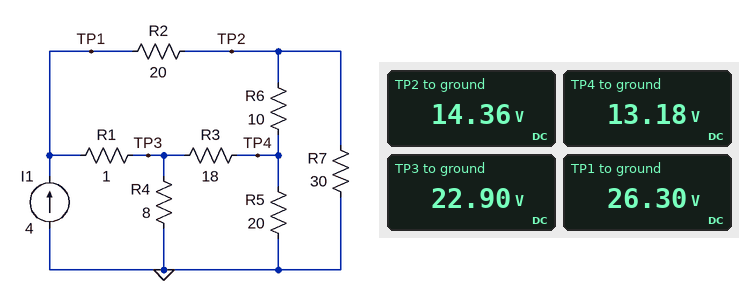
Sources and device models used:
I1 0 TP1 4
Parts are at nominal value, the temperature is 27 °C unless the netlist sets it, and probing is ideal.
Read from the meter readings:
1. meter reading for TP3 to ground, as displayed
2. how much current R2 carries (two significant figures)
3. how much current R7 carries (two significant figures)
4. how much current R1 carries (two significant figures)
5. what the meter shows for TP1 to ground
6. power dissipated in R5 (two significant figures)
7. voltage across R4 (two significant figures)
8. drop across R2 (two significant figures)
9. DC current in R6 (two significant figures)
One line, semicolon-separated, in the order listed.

22.90 V; 600 mA; 480 mA; 3.4 A; 26.30 V; 8.7 W; 23 V; 12 V; 120 mA
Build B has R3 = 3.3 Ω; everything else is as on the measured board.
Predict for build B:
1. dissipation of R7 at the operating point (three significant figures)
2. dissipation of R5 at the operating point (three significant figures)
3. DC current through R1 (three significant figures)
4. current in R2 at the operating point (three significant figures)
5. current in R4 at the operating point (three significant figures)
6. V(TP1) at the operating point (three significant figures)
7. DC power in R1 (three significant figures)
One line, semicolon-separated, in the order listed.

8.68 W; 15.2 W; 3.59 A; 409 mA; 2.59 A; 24.3 V; 12.9 W
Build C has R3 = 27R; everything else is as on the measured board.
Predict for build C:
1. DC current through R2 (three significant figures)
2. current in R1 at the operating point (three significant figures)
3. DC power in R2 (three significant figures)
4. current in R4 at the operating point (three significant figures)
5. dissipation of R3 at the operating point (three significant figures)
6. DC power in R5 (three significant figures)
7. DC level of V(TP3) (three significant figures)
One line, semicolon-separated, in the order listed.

646 mA; 3.35 A; 8.34 W; 2.93 A; 4.80 W; 7.29 W; 23.5 V
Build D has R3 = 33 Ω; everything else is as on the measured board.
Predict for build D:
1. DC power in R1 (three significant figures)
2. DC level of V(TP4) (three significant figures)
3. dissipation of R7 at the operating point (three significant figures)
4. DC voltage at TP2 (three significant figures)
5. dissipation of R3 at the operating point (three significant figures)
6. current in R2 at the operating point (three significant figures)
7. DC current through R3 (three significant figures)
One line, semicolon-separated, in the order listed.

11.1 W; 11.6 V; 6.25 W; 13.7 V; 4.46 W; 668 mA; 368 mA
